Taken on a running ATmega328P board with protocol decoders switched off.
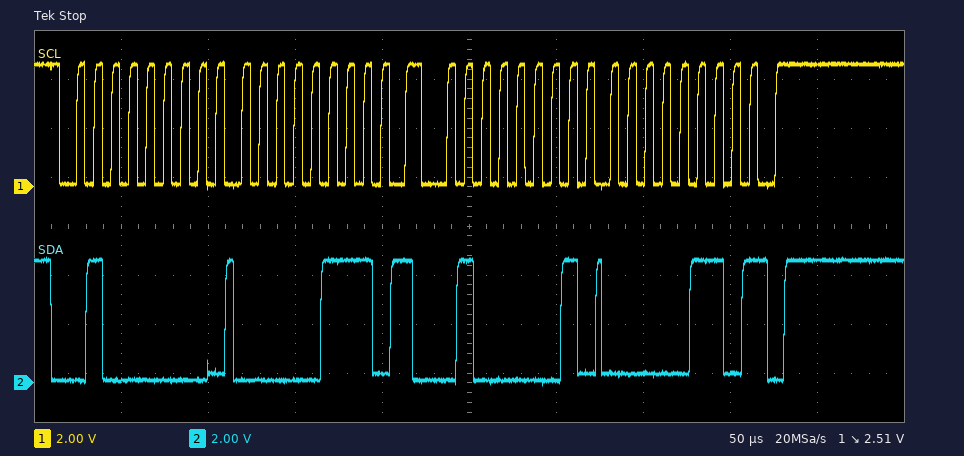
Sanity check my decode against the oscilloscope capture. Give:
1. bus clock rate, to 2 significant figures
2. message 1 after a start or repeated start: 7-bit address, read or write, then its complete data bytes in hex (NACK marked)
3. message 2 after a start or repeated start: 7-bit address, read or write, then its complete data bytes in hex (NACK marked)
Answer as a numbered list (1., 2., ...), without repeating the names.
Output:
1. 100 kHz
2. 0x20 write: 07
3. 0x20 read: 06 NACK
